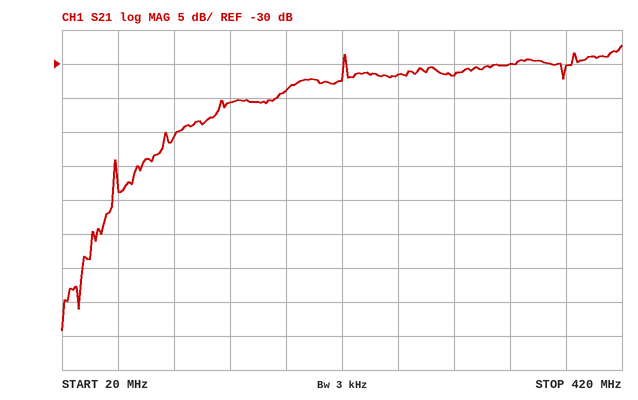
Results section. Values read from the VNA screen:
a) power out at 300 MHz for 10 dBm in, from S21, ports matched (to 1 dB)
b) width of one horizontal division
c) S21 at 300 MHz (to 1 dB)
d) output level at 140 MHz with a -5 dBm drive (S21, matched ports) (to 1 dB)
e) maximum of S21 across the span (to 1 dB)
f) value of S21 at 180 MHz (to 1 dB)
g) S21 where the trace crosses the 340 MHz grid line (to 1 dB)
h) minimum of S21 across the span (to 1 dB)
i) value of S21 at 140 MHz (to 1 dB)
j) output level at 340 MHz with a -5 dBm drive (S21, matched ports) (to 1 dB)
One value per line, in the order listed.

-22 dBm
40 MHz
-32 dB
-41 dBm
-27 dB
-34 dB
-30 dB
-69 dB
-36 dB
-35 dBm
